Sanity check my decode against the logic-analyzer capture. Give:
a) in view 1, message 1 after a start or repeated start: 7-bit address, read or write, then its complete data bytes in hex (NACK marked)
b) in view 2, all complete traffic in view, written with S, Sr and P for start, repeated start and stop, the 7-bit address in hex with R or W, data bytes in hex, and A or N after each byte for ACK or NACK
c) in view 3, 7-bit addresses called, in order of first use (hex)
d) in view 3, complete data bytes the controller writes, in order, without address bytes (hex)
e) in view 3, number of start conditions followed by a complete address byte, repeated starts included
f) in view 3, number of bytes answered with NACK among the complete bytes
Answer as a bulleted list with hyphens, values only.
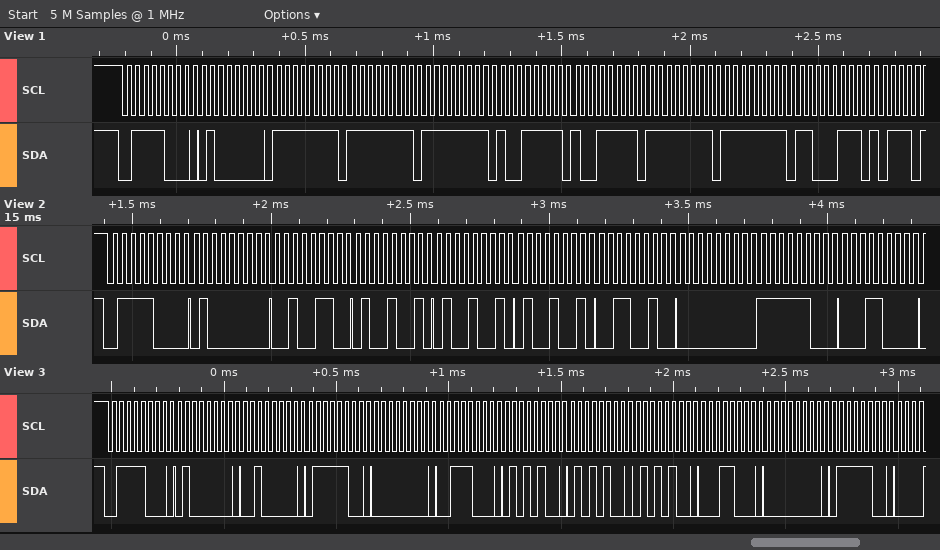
- 0x3C write: 40 FF FF FF 9F 9F FF FF C7
- S 3CW A 40 A 26 A 49 A 49 A 49 A 32 A 00 A FC A 18 A
- 0x3C
- 40 20 7C 00 38 54 54 54 18 00 7C
- 1
- 0
